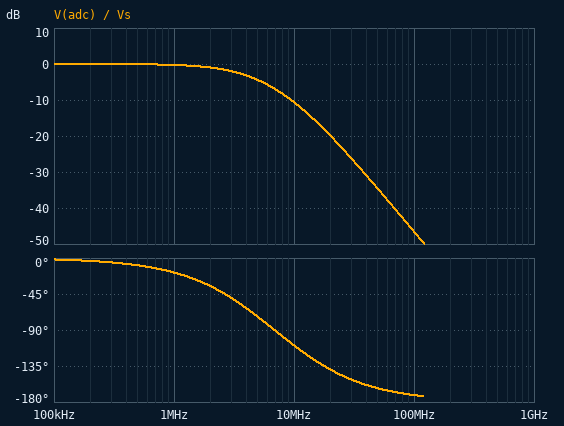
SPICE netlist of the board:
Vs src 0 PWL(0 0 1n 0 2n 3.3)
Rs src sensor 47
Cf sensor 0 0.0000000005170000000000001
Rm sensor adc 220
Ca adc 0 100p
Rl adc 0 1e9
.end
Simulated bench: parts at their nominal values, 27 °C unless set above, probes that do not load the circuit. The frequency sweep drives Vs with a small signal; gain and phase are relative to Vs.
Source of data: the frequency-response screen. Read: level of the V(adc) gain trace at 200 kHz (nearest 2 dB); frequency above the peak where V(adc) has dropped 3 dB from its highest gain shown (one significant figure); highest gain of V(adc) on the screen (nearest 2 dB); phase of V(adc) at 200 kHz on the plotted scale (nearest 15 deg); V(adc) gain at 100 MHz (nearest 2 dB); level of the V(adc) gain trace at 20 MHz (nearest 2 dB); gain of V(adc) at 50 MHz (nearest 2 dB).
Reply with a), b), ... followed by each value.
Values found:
a) 0 dB
b) 4 MHz
c) 0 dB
d) 0 deg
e) -46 dB
f) -20 dB
g) -34 dB
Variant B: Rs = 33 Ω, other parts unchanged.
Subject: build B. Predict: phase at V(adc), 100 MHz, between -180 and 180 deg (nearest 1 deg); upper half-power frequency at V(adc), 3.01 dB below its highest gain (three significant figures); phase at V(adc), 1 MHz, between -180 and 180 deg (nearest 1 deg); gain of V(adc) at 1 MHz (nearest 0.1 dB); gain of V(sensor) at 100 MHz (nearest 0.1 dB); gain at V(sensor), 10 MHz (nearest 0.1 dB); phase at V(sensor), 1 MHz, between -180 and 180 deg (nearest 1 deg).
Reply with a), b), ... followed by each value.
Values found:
a) -170 deg
b) 4.66 MHz
c) -15 deg
d) -0.2 dB
e) -20.7 dB
f) -4.0 dB
g) -7 deg
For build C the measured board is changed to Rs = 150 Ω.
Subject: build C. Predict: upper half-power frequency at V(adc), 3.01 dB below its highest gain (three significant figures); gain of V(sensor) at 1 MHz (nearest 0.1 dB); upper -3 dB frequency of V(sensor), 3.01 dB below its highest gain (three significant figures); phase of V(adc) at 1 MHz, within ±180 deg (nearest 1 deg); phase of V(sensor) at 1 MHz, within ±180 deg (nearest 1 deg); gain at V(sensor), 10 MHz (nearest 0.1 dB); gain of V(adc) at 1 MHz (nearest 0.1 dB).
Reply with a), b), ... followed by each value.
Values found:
a) 1.59 MHz
b) -1.3 dB
c) 1.67 MHz
d) -38 deg
e) -30 deg
f) -14.6 dB
g) -1.4 dB
